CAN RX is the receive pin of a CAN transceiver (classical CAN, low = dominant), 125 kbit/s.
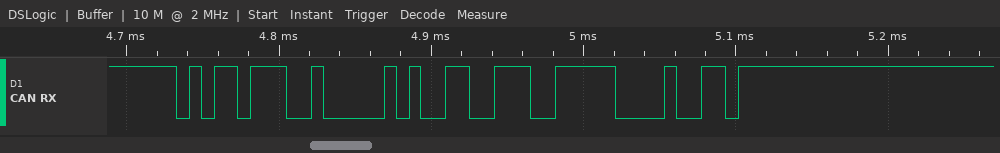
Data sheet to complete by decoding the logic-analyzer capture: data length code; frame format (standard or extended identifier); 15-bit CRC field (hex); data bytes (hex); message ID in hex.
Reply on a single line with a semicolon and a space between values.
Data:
1; standard; 0x4F89; 33; 0x5B9
